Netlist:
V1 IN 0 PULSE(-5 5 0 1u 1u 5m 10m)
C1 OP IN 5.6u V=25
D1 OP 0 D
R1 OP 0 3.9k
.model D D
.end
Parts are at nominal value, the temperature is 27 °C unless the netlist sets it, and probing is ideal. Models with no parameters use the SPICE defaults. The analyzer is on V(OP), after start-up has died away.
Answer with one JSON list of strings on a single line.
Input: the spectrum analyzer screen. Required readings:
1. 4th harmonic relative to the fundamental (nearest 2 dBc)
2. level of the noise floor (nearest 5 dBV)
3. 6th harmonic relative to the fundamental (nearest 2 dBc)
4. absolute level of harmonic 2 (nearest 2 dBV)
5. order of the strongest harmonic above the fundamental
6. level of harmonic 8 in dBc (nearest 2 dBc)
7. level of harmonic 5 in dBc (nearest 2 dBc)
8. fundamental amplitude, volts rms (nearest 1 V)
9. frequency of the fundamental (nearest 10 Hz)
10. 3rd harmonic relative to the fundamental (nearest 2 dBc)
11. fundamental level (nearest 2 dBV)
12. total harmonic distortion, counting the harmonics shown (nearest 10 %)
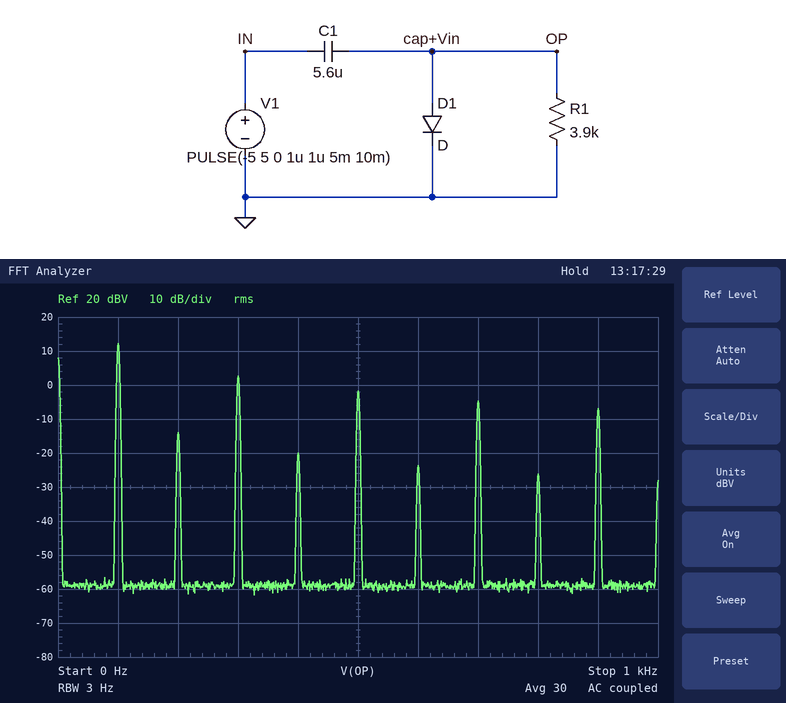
["-32 dBc", "-60 dBV", "-36 dBc", "-14 dBV", "3", "-38 dBc", "-14 dBc", "4 V", "100 Hz", "-10 dBc", "12 dBV", "40 %"]
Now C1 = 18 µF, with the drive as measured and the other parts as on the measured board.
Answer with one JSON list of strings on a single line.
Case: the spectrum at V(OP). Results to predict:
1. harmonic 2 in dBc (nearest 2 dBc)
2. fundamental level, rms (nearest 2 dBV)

["-36 dBc", "12 dBV"]
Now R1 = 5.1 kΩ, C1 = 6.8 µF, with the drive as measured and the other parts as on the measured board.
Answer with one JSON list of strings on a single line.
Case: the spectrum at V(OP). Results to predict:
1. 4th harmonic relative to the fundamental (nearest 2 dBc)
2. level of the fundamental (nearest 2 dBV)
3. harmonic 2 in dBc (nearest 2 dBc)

["-36 dBc", "12 dBV", "-30 dBc"]
